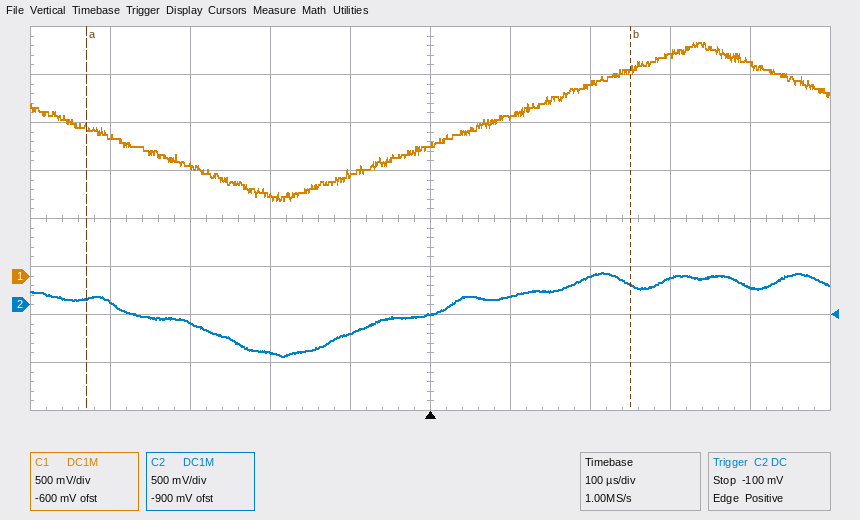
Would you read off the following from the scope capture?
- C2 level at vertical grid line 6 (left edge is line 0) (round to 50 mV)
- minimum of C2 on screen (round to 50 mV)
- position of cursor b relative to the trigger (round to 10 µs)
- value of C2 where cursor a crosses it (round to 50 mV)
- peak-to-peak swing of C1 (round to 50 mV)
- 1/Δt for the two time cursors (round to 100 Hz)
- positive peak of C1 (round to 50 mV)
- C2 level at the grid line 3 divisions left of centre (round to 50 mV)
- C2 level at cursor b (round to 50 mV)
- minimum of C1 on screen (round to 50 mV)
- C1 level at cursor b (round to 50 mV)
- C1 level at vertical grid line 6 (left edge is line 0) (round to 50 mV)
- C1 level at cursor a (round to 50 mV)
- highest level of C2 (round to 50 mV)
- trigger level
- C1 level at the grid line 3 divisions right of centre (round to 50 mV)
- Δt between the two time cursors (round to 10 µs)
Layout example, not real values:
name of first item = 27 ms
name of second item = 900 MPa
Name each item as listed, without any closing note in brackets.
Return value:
C2 level at vertical grid line 6 (left edge is line 0) = 100 mV
minimum of C2 on screen = -550 mV
position of cursor b relative to the trigger = +250 µs
value of C2 where cursor a crosses it = 50 mV
peak-to-peak swing of C1 = 1.65 V
1/Δt for the two time cursors = 1.5 kHz
positive peak of C1 = 2.45 V
C2 level at the grid line 3 divisions left of centre = -200 mV
C2 level at cursor b = 200 mV
minimum of C1 on screen = 800 mV
C1 level at cursor b = 2.15 V
C1 level at vertical grid line 6 (left edge is line 0) = 1.65 V
C1 level at cursor a = 1.55 V
highest level of C2 = 350 mV
trigger level = -100 mV
C1 level at the grid line 3 divisions right of centre = 2.30 V
Δt between the two time cursors = 680 µs
